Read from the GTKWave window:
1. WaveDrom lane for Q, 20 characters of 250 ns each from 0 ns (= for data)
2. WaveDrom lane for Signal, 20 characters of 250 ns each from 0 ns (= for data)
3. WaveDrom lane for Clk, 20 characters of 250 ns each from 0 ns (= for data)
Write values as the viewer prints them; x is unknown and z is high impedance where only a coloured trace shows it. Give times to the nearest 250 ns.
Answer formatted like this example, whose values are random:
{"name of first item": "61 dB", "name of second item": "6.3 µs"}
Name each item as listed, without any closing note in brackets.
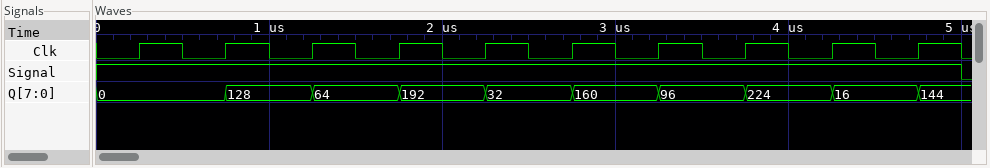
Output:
{"WaveDrom lane for Q, 20 characters of 250 ns each from 0 ns": "{name: 'Q', wave: '=..=.=.=.=.=.=.=.=.=', data: '0 128 64 192 32 160 96 224 16 144'}", "WaveDrom lane for Signal, 20 characters of 250 ns each from 0 ns": "{name: 'Signal', wave: '1...................'}", "WaveDrom lane for Clk, 20 characters of 250 ns each from 0 ns": "{name: 'Clk', wave: '01010101010101010101'}"}
